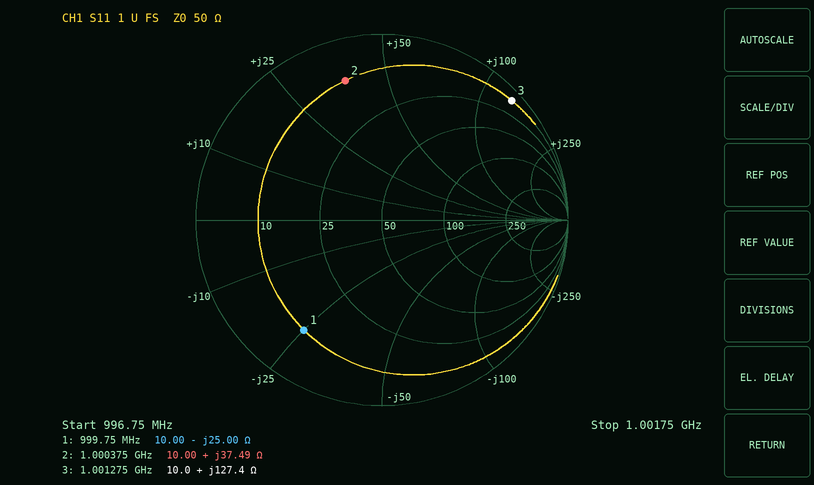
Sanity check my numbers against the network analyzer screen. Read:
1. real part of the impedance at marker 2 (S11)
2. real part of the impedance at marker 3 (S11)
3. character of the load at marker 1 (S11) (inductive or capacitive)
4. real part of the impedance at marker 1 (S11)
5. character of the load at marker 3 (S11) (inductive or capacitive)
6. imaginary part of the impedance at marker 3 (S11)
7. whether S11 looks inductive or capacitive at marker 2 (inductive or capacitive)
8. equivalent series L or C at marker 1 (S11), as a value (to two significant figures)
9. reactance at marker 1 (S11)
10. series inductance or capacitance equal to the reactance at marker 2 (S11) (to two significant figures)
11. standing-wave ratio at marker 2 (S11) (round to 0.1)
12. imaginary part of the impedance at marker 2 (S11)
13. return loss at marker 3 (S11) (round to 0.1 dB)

10.00 Ω
10.0 Ω
capacitive
10.00 Ω
inductive
+127.4 Ω
inductive
6.4 pF
-25.00 Ω
6.0 nH
7.9
+37.49 Ω
0.5 dB
